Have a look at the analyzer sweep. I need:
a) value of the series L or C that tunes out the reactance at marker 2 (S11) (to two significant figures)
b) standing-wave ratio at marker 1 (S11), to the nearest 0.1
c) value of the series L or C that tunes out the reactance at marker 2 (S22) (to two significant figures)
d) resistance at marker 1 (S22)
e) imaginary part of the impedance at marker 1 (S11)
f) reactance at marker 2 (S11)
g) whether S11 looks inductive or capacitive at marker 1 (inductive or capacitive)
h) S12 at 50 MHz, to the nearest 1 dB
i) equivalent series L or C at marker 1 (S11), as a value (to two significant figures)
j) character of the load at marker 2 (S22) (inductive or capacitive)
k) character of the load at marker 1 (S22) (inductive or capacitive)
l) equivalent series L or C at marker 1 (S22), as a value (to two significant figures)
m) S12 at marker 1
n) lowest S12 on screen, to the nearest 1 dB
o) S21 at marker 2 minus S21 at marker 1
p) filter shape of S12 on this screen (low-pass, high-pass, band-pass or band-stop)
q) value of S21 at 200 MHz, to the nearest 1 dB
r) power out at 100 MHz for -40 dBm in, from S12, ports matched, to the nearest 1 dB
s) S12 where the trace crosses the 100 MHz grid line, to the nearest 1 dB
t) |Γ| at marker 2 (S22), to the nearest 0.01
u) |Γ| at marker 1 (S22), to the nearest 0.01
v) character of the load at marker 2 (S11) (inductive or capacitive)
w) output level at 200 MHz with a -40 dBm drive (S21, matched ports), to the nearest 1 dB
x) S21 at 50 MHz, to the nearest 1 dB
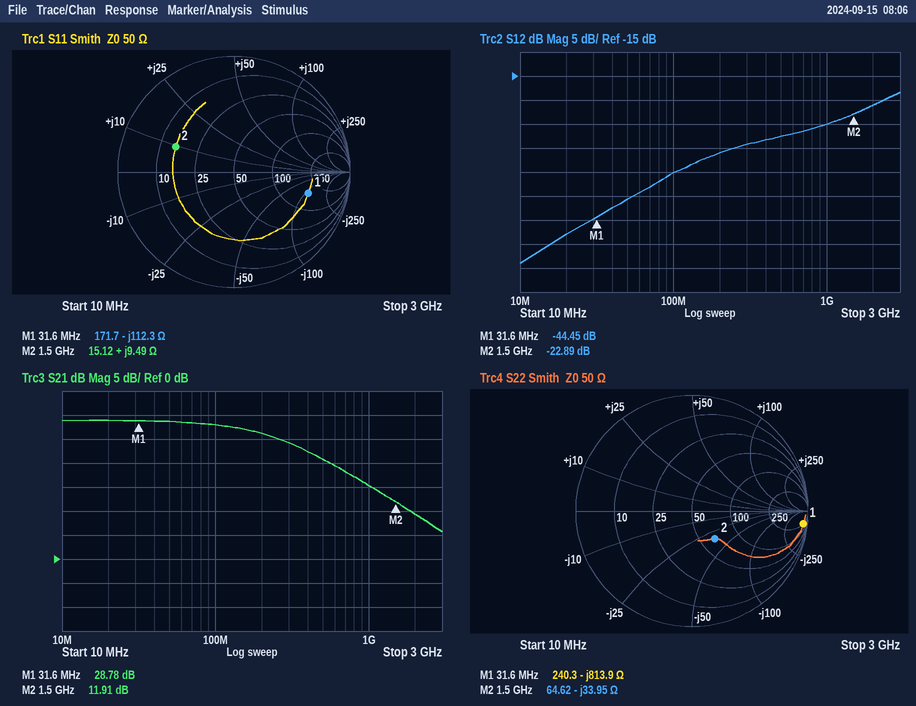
11 pF
5.0
3.6 nH
240.3 Ω
-112.3 Ω
+9.49 Ω
capacitive
-41 dB
45 pF
capacitive
capacitive
6.2 pF
-44.45 dB
-54 dB
-16.87 dB
high-pass
26 dB
-75 dBm
-35 dB
0.31
0.97
inductive
-14 dBm
29 dB
